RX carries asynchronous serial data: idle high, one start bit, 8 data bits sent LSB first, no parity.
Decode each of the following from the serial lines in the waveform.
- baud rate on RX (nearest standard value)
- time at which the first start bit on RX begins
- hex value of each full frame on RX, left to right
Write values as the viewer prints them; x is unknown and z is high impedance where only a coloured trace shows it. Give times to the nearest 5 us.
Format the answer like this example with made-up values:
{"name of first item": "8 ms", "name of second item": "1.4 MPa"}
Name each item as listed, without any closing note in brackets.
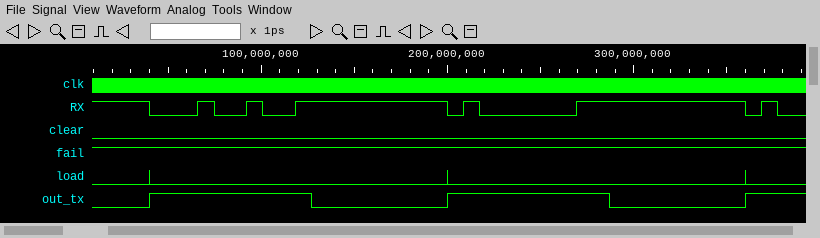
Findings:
{"baud rate on RX": "115200 baud", "time at which the first start bit on RX begins": "40 us", "hex value of each full frame on RX, left to right": "24, 81"}
